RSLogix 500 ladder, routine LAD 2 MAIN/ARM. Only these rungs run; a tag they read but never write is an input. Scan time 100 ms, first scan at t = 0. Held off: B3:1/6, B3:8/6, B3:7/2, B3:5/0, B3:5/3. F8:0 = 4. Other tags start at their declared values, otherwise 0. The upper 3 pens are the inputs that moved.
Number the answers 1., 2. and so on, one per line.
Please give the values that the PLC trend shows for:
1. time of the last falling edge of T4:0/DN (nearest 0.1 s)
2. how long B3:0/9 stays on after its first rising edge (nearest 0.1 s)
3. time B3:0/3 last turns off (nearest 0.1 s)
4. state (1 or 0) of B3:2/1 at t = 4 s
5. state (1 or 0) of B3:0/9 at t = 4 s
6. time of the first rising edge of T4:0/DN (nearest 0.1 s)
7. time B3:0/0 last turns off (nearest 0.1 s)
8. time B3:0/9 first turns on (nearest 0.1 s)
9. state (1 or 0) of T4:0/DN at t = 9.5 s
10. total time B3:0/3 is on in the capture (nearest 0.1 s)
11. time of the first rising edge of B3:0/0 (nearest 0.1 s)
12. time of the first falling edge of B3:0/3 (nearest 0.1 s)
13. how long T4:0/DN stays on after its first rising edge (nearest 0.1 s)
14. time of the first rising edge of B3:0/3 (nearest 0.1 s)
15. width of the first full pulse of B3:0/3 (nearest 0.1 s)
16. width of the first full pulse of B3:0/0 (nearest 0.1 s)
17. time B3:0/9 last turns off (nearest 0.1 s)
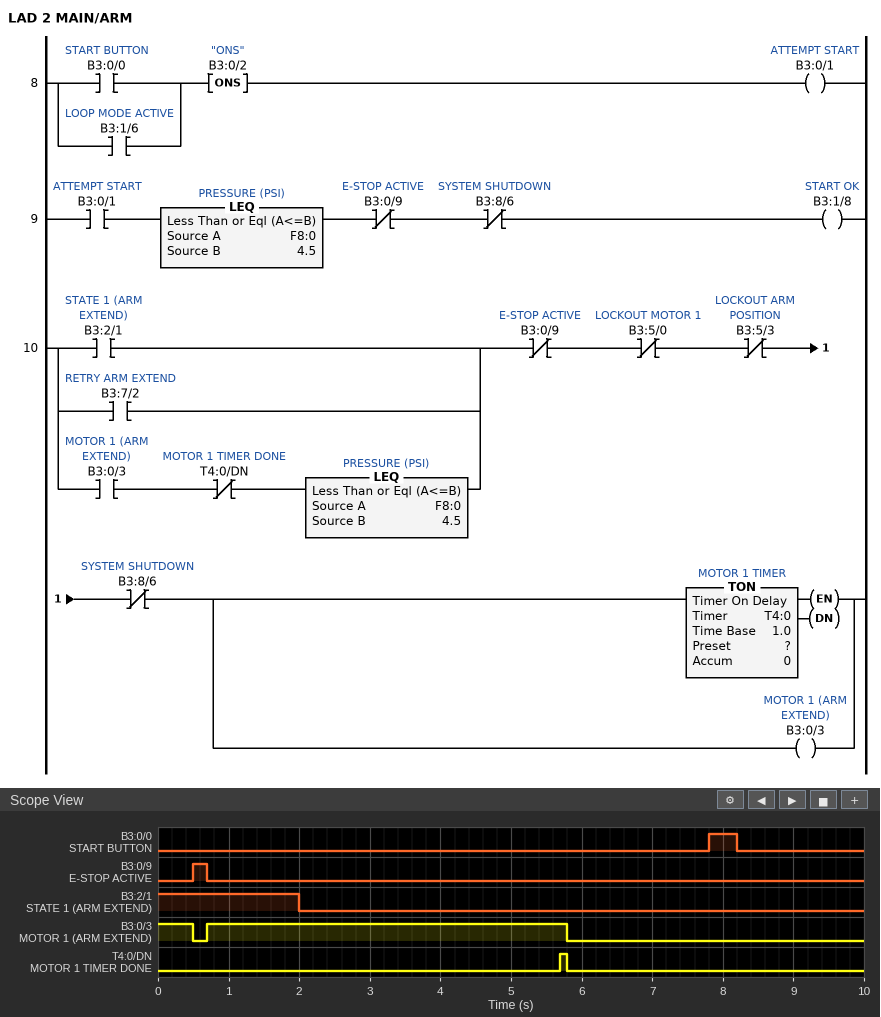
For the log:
1. 5.8 s
2. 0.2 s
3. 5.8 s
4. 0
5. 0
6. 5.7 s
7. 8.2 s
8. 0.5 s
9. 0
10. 5.6 s
11. 7.8 s
12. 0.5 s
13. 0.1 s
14. 0.7 s
15. 5.1 s
16. 0.4 s
17. 0.7 s
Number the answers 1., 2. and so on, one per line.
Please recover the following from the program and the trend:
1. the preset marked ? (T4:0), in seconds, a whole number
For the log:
1. 5 s
